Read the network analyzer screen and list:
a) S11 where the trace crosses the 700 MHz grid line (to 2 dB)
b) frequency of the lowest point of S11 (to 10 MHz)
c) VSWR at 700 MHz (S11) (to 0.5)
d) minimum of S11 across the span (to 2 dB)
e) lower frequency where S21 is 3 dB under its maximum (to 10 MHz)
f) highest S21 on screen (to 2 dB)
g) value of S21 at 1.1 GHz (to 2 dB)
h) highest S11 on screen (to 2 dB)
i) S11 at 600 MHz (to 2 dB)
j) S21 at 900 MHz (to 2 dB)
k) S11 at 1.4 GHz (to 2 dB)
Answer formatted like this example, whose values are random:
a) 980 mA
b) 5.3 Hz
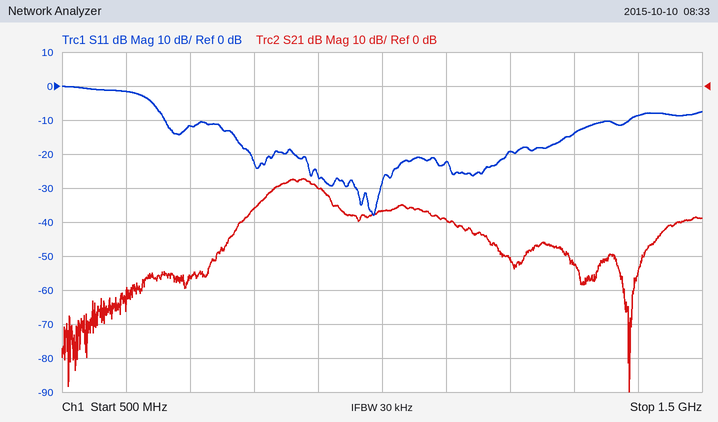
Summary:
a) -12 dB
b) 990 MHz
c) 1.5
d) -38 dB
e) 830 MHz
f) -28 dB
g) -40 dB
h) 0 dB
i) -2 dB
j) -30 dB
k) -8 dB
